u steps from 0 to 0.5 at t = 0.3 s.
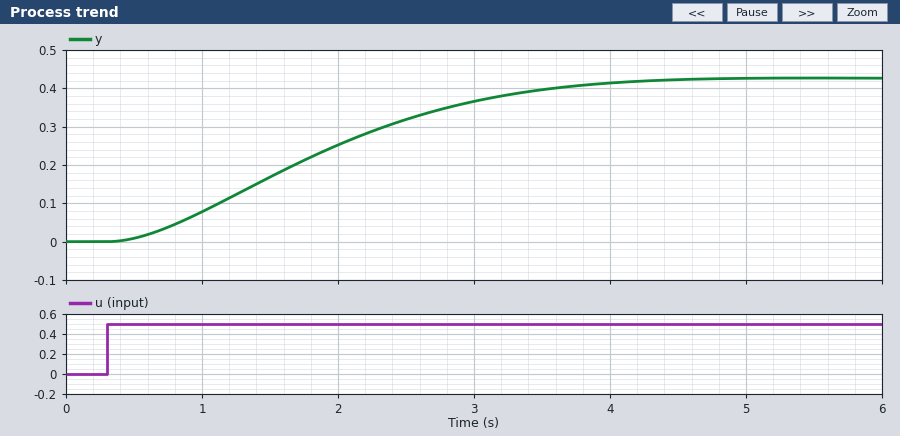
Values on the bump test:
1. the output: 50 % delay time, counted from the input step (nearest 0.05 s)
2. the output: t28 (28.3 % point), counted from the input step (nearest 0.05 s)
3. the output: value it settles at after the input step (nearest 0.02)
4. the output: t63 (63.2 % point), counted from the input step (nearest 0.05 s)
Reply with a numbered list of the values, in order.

1. 1.45 s
2. 0.95 s
3. 0.42
4. 1.80 s
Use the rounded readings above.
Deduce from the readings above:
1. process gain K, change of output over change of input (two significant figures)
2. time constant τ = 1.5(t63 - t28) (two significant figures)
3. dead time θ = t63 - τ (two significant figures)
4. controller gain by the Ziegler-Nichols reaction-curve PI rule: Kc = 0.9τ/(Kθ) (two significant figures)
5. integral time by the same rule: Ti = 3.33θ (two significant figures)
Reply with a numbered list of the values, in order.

1. 0.84
2. 1.3 s
3. 0.50 s
4. 2.8
5. 1.7 s
